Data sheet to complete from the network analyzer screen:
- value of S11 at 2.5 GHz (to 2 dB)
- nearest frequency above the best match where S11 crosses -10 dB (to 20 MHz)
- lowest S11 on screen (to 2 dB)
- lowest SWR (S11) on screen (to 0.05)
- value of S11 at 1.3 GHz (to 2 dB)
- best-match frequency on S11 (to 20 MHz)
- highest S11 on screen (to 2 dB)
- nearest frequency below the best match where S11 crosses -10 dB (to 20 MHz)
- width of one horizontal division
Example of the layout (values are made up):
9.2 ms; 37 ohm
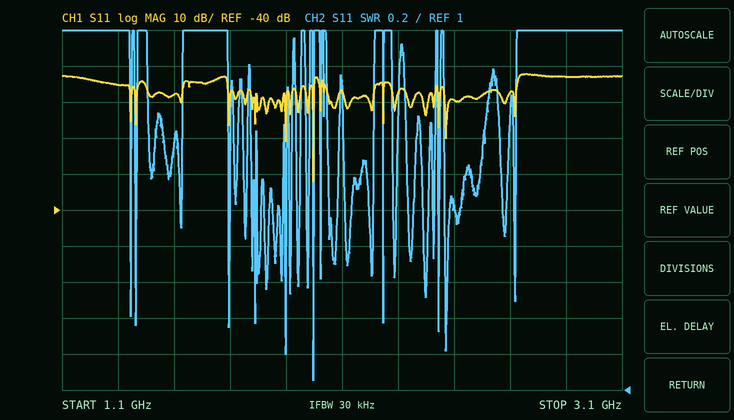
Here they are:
-10 dB; 2.00 GHz; -32 dB; 1.05; -6 dB; 2.00 GHz; -2 dB; 2.00 GHz; 200 MHz
